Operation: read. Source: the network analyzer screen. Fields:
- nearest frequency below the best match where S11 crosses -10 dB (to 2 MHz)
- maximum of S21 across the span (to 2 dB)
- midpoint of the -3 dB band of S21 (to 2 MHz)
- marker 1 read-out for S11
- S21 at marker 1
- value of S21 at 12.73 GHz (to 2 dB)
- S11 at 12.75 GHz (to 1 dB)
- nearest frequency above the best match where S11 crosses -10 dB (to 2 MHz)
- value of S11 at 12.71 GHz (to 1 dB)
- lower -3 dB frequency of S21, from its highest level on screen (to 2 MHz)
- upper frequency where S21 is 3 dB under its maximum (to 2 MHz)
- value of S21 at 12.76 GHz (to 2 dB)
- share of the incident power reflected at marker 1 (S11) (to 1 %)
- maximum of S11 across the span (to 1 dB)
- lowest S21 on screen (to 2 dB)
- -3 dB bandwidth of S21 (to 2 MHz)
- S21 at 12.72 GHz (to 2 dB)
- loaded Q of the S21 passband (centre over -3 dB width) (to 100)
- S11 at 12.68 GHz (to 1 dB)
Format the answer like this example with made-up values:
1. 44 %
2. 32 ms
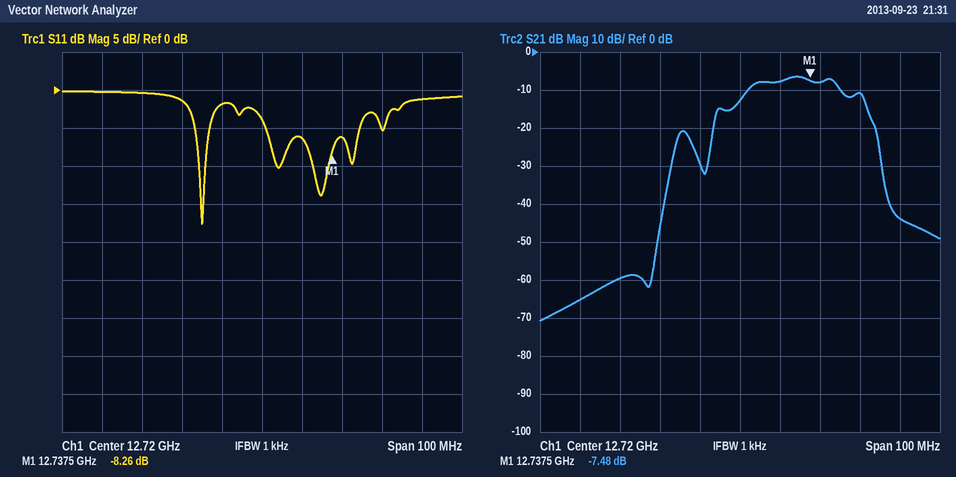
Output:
1. 12.704 GHz
2. -6 dB
3. 12.734 GHz
4. -8.26 dB
5. -7.48 dB
6. -8 dB
7. -5 dB
8. 12.706 GHz
9. -2 dB
10. 12.722 GHz
11. 12.744 GHz
12. -44 dB
13. 15 %
14. 0 dB
15. -70 dB
16. 22 MHz
17. -12 dB
18. 600
19. 0 dB
